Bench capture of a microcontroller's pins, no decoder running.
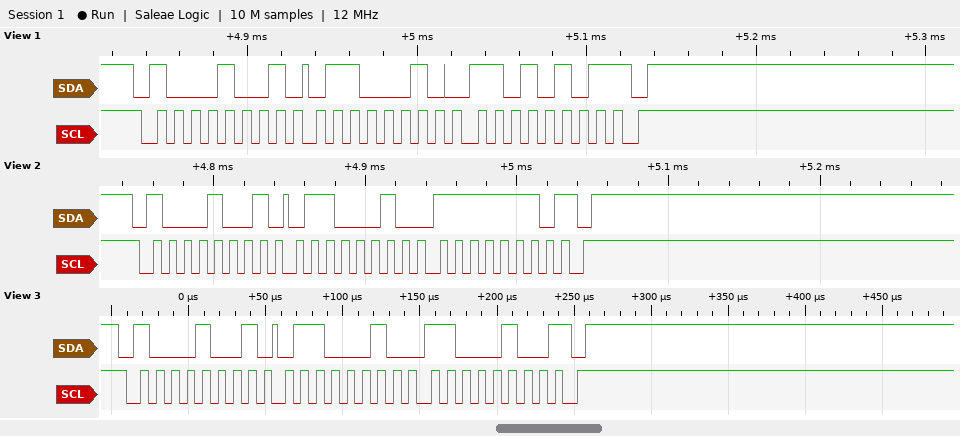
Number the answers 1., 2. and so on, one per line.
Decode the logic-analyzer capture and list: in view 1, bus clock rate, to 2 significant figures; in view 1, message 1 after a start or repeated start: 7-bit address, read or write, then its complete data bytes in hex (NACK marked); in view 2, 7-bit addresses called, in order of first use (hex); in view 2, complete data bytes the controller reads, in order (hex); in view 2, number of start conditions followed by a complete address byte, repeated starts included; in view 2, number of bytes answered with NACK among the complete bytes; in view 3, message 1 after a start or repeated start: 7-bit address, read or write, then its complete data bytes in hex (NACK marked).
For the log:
1. 100 kHz
2. 0x44 read: 62 D5 NACK
3. 0x44
4. 62 FE
5. 1
6. 1
7. 0x44 read: 62 C4 NACK
